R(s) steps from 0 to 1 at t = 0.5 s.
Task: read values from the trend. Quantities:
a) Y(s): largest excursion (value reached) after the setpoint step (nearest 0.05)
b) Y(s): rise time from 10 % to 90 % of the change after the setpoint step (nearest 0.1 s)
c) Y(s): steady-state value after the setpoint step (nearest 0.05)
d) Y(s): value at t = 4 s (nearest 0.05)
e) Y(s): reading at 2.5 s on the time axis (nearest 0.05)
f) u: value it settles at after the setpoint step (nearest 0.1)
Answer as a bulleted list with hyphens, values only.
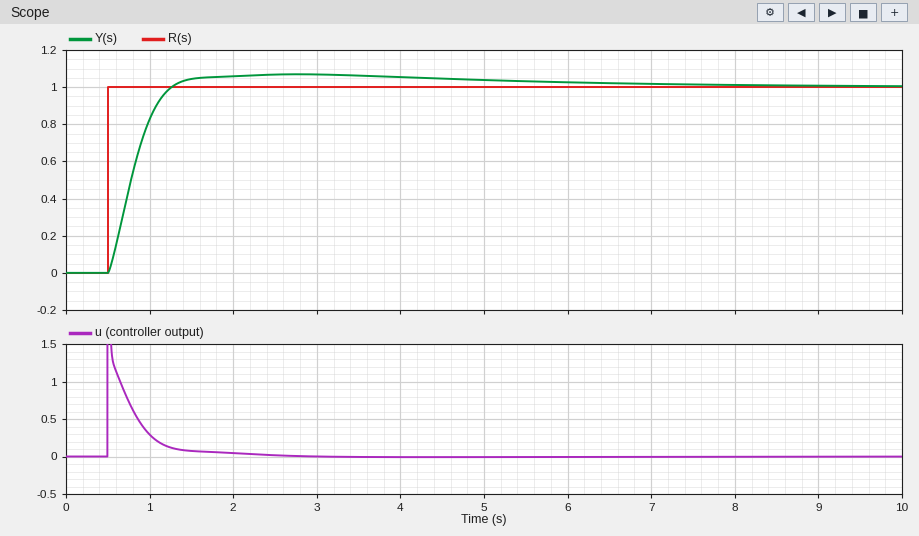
- 1.05
- 0.5 s
- 1.00
- 1.05
- 1.05
- 0.0
